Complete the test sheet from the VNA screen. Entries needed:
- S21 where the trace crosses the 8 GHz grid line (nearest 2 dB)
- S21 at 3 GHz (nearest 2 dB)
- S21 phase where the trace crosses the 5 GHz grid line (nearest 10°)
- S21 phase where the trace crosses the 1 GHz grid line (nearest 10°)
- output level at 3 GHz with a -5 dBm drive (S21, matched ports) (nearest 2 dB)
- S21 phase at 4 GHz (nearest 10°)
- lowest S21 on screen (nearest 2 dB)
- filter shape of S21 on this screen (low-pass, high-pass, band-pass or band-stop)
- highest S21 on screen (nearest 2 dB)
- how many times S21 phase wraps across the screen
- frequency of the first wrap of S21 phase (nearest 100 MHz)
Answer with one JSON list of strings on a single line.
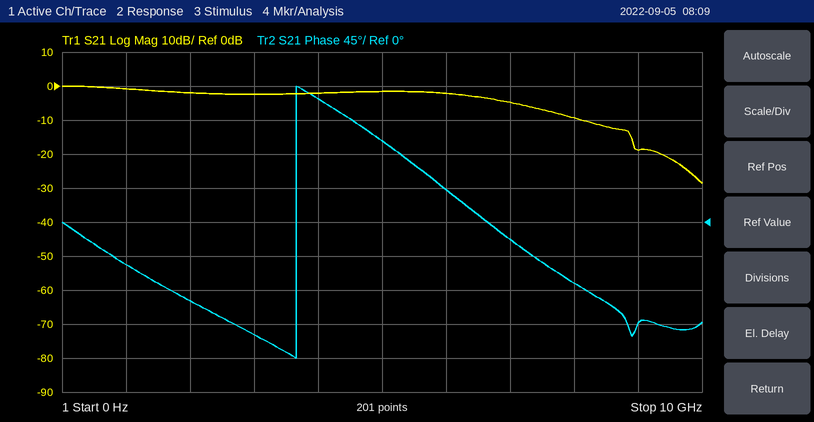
["-10 dB", "-2 dB", "110°", "-60°", "-8 dBm", "160°", "-28 dB", "low-pass", "0 dB", "1", "3.7 GHz"]
